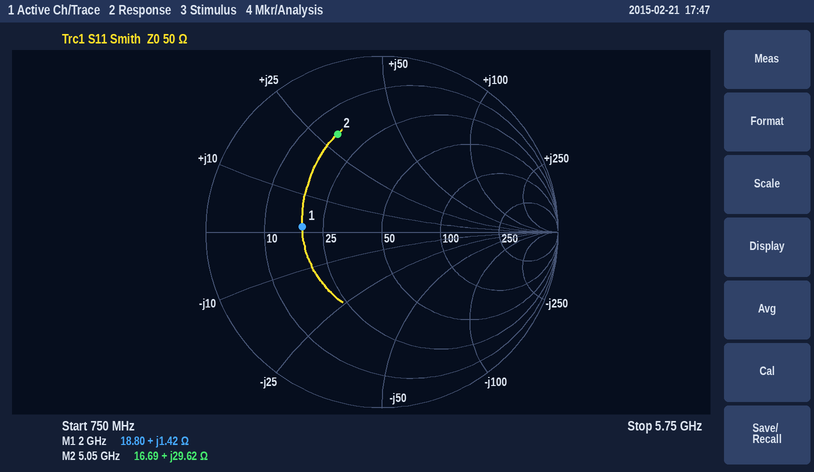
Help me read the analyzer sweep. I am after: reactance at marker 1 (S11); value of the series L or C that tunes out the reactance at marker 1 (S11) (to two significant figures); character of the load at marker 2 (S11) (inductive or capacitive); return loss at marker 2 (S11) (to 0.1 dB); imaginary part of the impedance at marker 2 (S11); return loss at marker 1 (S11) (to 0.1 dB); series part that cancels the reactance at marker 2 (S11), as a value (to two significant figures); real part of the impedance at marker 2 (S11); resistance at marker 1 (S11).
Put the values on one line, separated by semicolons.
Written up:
+1.42 Ω; 56 pF; inductive; 4.3 dB; +29.62 Ω; 6.9 dB; 1.1 pF; 16.69 Ω; 18.80 Ω
